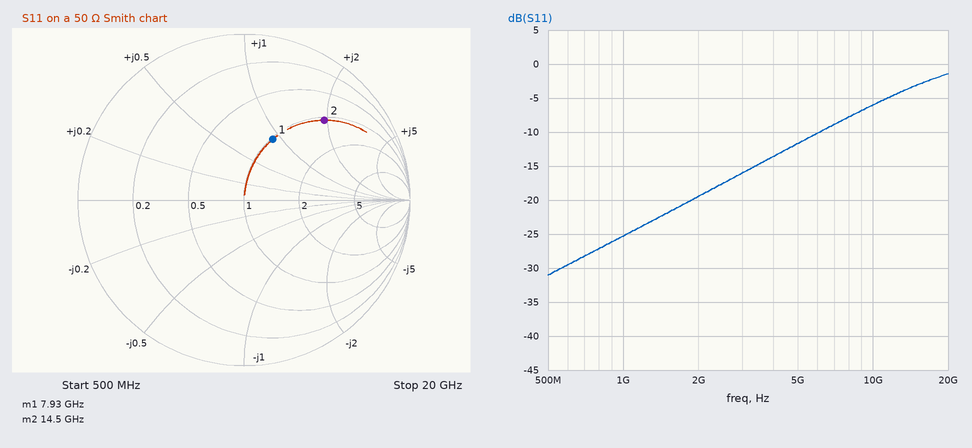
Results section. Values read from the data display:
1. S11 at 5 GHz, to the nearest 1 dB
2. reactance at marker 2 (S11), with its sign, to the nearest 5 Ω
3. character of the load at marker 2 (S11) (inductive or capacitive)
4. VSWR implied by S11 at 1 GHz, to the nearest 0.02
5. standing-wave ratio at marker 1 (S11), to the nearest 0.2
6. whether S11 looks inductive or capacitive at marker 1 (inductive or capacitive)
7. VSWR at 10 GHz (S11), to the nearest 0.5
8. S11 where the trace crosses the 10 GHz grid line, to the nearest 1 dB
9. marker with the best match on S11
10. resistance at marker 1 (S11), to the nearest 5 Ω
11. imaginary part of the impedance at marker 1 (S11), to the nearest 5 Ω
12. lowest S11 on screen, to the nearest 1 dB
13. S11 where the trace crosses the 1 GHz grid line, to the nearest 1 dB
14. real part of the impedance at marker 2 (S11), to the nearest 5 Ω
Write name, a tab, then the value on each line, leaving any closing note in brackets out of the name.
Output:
S11 at 5 GHz, to the nearest 1 dB	-12 dB
reactance at marker 2 (S11), with its sign, to the nearest 5 Ω	+95 Ω
character of the load at marker 2 (S11)	inductive
VSWR implied by S11 at 1 GHz, to the nearest 0.02	1.12
standing-wave ratio at marker 1 (S11), to the nearest 0.2	2.4
whether S11 looks inductive or capacitive at marker 1	inductive
VSWR at 10 GHz (S11), to the nearest 0.5	3.0
S11 where the trace crosses the 10 GHz grid line, to the nearest 1 dB	-6 dB
marker with the best match on S11	marker 1
resistance at marker 1 (S11), to the nearest 5 Ω	50 Ω
imaginary part of the impedance at marker 1 (S11), to the nearest 5 Ω	+45 Ω
lowest S11 on screen, to the nearest 1 dB	-31 dB
S11 where the trace crosses the 1 GHz grid line, to the nearest 1 dB	-25 dB
real part of the impedance at marker 2 (S11), to the nearest 5 Ω	55 Ω
